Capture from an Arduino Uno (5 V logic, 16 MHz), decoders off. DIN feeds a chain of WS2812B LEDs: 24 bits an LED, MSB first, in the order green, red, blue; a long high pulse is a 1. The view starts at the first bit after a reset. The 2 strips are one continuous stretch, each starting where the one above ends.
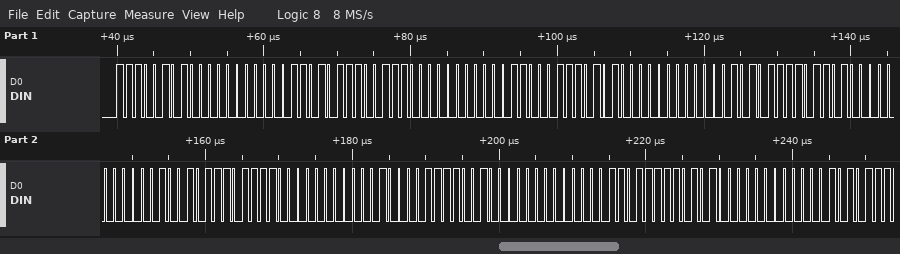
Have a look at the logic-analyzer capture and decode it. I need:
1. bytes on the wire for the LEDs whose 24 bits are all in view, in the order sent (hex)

E5 00 1A E7 00 18 EA 00 15 ED 00 12 EF 00 10 F2 00 0D F5 00 0A
